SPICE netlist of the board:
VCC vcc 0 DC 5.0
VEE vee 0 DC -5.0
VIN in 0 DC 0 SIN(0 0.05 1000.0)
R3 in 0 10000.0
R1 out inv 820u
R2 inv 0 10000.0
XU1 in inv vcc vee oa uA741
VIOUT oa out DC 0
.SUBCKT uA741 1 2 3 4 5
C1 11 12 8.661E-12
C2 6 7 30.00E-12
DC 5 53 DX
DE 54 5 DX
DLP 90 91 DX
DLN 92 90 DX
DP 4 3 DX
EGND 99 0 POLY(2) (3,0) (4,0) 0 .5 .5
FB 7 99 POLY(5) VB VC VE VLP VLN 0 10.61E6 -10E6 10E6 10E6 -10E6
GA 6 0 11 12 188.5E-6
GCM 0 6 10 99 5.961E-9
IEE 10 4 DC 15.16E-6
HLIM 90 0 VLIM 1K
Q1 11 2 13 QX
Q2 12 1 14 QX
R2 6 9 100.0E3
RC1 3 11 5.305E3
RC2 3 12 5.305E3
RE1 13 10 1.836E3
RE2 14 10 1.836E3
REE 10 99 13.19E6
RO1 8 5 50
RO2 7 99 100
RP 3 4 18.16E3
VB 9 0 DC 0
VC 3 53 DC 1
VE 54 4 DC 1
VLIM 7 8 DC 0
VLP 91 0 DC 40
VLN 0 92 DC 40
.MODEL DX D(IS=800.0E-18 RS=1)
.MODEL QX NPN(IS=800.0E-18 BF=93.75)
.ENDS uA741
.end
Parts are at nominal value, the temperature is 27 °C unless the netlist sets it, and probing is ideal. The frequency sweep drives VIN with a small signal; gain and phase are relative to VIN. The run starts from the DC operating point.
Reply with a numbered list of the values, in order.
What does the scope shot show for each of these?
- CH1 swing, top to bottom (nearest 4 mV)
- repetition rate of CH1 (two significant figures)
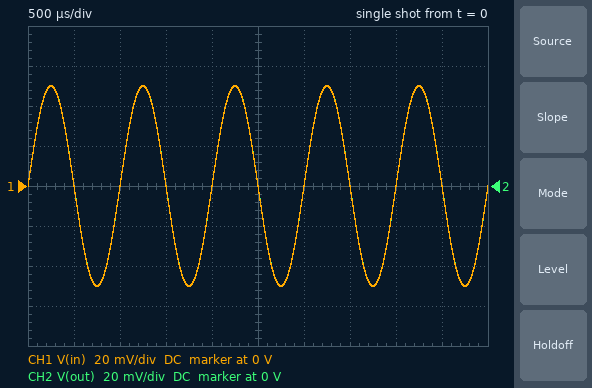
1. 100 mV
2. 1.0 kHz
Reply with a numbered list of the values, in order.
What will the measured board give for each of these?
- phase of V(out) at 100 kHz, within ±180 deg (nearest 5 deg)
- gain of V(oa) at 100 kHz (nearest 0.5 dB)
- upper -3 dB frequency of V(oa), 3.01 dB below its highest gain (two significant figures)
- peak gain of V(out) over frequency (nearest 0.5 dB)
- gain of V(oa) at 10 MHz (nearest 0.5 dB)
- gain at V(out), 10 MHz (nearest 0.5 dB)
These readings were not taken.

1. -5 deg
2. 0 dB
3. 1.4 MHz
4. 0 dB
5. -35.5 dB
6. -35.5 dB
